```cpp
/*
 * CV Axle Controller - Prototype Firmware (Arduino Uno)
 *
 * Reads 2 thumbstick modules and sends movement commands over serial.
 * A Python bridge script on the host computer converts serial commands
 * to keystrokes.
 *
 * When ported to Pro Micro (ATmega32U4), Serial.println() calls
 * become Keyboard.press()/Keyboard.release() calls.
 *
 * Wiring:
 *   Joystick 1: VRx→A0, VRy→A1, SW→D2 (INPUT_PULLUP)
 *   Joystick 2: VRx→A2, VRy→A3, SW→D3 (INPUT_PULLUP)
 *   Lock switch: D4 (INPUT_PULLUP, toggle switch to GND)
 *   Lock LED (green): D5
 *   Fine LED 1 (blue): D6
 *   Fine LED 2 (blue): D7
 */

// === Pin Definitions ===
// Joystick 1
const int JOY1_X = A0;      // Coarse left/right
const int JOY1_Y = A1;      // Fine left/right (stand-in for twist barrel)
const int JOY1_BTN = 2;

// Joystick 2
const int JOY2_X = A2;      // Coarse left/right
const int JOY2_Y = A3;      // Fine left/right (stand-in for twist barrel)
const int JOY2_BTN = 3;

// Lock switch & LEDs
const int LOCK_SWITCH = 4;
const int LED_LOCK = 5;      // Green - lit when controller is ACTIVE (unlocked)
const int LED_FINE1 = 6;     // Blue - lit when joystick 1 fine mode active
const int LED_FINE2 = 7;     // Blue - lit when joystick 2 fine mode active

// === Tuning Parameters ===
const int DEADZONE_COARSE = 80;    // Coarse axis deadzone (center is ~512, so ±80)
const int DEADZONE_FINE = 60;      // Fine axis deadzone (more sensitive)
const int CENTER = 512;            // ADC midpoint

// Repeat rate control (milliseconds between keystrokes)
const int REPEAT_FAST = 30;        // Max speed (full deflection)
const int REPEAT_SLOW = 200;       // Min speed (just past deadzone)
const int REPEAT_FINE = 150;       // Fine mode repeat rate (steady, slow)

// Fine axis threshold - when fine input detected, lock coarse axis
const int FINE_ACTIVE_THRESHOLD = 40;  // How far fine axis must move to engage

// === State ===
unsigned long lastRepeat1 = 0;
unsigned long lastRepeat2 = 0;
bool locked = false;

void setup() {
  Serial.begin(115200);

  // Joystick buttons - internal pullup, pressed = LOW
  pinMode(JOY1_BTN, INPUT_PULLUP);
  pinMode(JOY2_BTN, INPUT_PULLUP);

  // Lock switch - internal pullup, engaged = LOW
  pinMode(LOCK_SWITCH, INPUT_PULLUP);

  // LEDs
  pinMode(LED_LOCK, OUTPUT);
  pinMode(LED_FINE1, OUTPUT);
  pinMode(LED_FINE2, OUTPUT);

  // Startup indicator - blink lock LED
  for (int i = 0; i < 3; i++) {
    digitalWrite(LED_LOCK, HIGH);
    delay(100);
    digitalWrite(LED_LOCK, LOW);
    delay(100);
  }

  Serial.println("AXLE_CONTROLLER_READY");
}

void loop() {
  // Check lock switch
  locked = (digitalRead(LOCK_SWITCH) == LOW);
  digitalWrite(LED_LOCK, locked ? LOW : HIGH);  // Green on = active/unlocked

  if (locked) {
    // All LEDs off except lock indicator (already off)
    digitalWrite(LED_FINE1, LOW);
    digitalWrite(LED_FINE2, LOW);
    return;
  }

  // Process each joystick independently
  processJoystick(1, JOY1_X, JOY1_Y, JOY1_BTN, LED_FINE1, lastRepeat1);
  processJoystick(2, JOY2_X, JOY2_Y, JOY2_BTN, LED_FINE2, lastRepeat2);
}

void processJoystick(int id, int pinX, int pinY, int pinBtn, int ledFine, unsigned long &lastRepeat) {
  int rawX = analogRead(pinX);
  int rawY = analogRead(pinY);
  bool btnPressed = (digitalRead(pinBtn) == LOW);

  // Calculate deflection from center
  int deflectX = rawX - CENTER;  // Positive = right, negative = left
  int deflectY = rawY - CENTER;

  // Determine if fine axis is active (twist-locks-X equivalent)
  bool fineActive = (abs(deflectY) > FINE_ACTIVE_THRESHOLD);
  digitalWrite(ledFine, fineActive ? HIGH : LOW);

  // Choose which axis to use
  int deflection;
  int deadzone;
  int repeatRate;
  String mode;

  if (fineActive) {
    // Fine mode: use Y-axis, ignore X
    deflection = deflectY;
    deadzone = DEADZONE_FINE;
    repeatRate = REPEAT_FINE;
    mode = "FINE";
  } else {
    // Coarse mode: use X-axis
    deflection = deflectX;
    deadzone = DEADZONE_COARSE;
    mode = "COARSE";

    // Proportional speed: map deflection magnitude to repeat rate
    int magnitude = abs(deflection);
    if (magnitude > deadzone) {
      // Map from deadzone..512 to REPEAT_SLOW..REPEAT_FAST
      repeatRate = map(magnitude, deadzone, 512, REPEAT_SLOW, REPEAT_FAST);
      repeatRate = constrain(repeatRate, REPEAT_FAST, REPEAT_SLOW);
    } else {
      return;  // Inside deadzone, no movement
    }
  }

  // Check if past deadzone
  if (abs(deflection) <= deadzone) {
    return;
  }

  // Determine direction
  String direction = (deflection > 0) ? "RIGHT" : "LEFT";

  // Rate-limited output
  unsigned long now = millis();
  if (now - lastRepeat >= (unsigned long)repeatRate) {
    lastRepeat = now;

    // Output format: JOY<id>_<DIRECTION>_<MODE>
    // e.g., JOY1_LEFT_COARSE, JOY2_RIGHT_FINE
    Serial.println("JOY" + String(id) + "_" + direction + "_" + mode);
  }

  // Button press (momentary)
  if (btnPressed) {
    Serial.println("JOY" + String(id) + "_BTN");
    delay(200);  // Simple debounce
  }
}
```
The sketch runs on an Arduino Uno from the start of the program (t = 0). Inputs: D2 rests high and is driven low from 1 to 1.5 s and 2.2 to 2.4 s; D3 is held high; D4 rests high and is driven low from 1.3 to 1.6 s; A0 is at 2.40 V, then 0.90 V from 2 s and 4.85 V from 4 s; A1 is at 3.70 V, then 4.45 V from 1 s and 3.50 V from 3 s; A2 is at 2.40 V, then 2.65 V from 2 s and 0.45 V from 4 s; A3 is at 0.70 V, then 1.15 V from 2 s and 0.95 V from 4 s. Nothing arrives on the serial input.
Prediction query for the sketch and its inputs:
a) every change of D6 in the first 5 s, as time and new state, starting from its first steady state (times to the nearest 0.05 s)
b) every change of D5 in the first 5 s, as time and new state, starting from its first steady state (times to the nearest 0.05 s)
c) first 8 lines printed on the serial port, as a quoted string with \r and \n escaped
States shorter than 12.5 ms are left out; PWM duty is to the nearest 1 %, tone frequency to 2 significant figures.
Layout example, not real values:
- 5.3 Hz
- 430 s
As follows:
- 0 s low; 0.6 s high; 1.4 s low; 1.6 s high
- 0 s high; 0.1 s low; 0.2 s high; 0.3 s low; 0.4 s high; 0.5 s low; 0.6 s high; 1.4 s low; 1.6 s high
- "AXLE_CONTROLLER_READY\r\nJOY1_RIGHT_FINE\r\nJOY2_LEFT_FINE\r\nJOY1_RIGHT_FINE\r\nJOY2_LEFT_FINE\r\nJOY1_RIGHT_FINE\r\nJOY2_LEFT_FINE\r\nJOY1_BTN\r\n"
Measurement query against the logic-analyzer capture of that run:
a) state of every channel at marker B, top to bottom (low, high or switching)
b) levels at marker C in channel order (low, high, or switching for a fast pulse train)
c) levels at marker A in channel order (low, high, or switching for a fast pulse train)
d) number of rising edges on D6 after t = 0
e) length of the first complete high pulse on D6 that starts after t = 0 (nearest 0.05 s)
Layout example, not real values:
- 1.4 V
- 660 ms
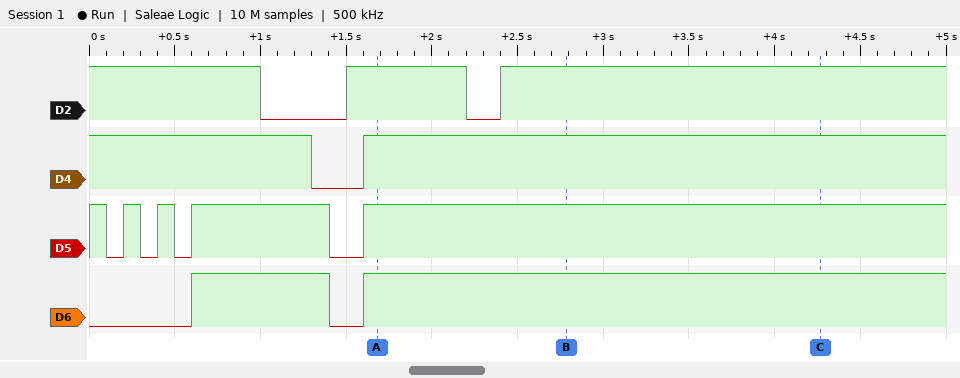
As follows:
- D2 high, D4 high, D5 high, D6 high
- D2 high, D4 high, D5 high, D6 high
- D2 high, D4 high, D5 high, D6 high
- 2
- 0.80 s
